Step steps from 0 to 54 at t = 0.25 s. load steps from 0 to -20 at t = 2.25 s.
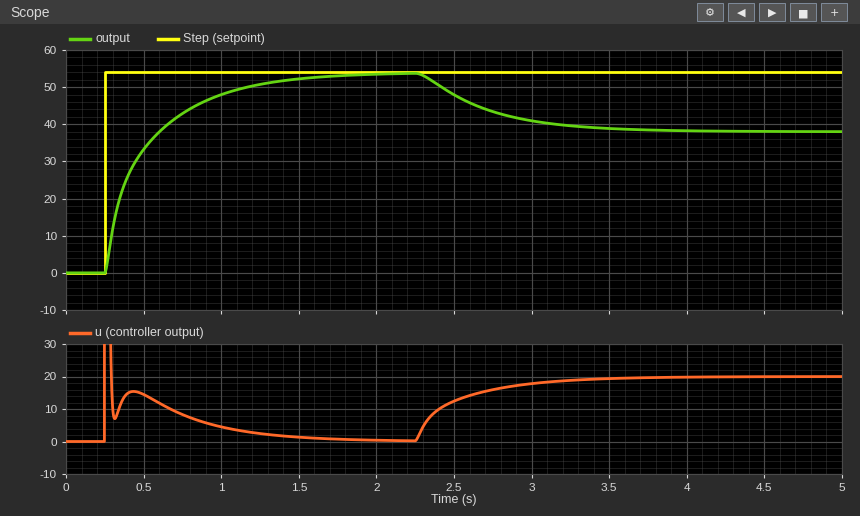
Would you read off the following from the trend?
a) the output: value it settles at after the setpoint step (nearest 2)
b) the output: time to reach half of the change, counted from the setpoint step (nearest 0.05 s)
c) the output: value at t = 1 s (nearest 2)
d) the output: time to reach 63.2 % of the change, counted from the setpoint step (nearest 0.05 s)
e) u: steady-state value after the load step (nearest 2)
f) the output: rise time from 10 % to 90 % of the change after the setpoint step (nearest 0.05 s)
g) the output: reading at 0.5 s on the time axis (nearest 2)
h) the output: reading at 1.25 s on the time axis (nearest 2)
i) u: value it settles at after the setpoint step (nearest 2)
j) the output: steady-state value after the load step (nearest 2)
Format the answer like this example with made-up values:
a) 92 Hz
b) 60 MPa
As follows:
a) 54
b) 0.15 s
c) 48
d) 0.25 s
e) 20
f) 0.75 s
g) 34
h) 50
i) 0
j) 38
